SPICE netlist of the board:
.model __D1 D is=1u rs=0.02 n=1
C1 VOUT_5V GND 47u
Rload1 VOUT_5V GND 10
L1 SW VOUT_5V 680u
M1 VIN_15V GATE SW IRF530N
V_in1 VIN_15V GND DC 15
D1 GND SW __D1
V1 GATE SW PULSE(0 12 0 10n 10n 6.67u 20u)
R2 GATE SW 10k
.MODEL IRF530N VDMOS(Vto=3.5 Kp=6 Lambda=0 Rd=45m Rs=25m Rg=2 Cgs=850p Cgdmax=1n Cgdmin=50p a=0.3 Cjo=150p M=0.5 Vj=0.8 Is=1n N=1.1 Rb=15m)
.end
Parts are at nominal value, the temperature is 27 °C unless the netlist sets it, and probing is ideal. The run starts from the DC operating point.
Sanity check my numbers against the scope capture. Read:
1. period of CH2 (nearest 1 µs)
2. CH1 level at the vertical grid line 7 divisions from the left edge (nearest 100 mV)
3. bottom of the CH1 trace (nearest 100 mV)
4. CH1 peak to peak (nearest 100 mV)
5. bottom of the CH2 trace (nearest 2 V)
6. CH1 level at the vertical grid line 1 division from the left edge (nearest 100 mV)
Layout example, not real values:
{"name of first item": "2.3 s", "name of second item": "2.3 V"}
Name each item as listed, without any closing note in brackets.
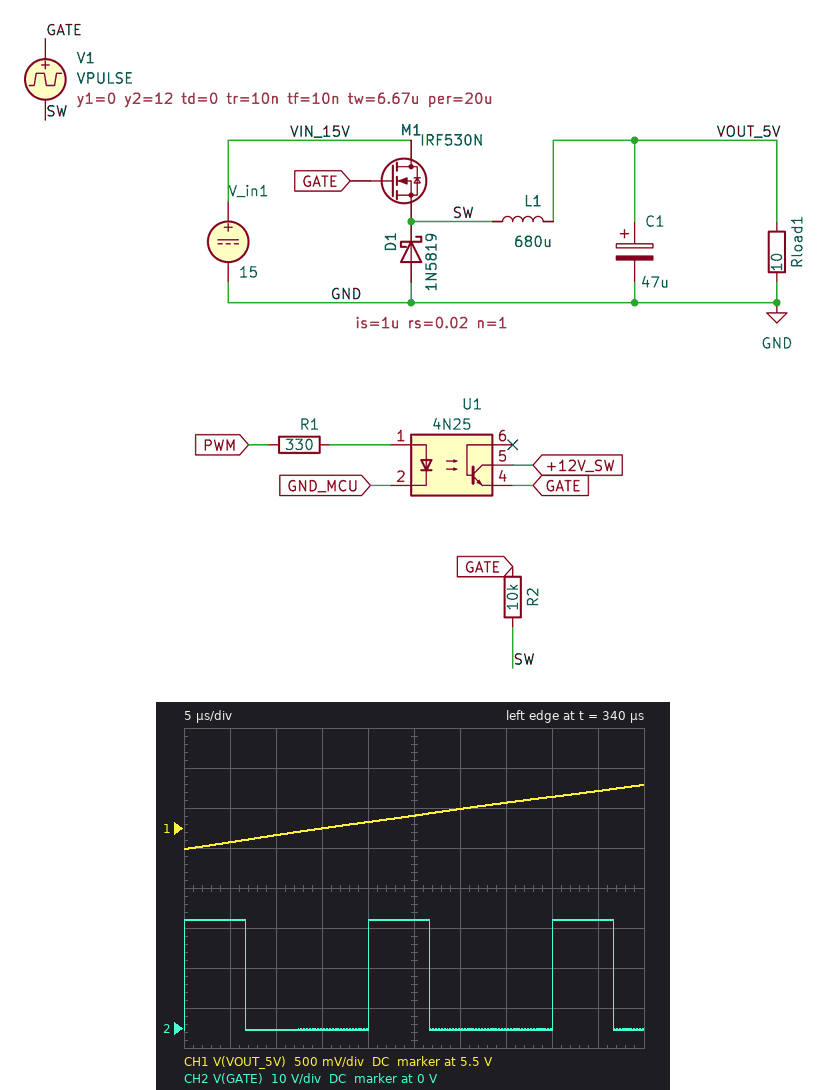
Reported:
{"period of CH2": "20 µs", "CH1 level at the vertical grid line 7 divisions from the left edge": "5.8 V", "bottom of the CH1 trace": "5.2 V", "CH1 peak to peak": "800 mV", "bottom of the CH2 trace": "0 V", "CH1 level at the vertical grid line 1 division from the left edge": "5.3 V"}
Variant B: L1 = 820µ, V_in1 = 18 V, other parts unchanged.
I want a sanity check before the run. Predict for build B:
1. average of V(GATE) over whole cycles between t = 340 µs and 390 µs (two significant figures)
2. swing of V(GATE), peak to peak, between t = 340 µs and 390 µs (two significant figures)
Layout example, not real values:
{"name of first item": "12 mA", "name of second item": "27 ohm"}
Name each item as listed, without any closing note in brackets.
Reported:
{"average of V(GATE) over whole cycles between t = 340 µs and 390 µs": "9.7 V", "swing of V(GATE), peak to peak, between t = 340 µs and 390 µs": "30 V"}
